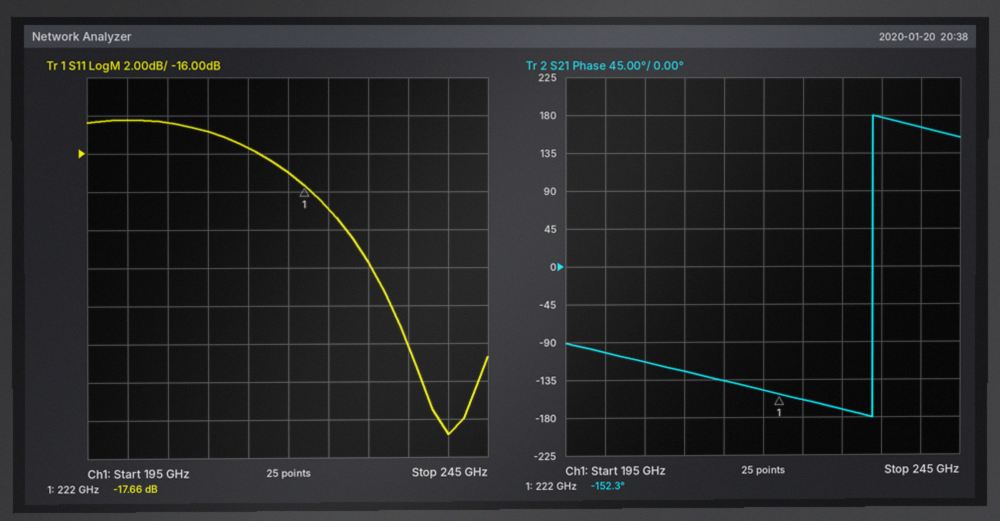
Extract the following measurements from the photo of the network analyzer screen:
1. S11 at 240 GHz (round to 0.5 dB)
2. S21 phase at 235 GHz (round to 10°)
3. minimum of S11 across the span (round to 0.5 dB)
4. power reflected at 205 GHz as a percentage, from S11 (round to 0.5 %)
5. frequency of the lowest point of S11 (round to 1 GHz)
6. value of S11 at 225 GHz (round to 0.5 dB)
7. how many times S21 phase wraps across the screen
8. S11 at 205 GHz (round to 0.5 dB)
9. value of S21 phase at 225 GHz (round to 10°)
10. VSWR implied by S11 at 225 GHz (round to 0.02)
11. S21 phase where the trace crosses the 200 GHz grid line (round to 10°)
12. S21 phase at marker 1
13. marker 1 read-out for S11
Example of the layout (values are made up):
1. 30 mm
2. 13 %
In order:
1. -31.0 dB
2. 180°
3. -31.0 dB
4. 3.5 %
5. 240 GHz
6. -19.0 dB
7. 1
8. -14.5 dB
9. -160°
10. 1.26
11. -100°
12. -152.3°
13. -17.66 dB
